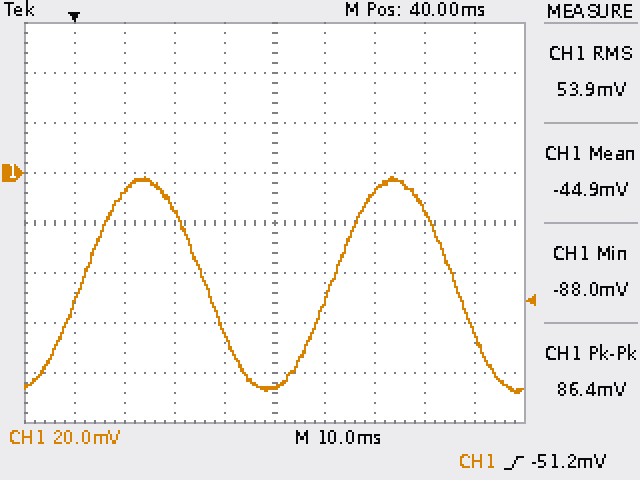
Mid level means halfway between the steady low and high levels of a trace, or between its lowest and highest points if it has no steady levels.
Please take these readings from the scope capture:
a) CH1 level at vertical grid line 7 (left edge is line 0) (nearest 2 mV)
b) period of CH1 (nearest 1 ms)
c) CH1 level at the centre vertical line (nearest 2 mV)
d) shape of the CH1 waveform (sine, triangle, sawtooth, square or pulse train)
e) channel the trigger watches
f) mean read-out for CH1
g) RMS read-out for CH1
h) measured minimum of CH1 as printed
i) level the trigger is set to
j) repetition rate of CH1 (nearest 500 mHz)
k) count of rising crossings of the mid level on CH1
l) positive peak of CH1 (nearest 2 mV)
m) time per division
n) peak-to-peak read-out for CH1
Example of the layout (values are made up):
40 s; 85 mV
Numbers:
-8 mV; 50 ms; -86 mV; sine; CH1; -44.9 mV; 53.9 mV; -88.0 mV; -51.2 mV; 20.0 Hz; 2; -2 mV; 10 ms; 86.4 mV
